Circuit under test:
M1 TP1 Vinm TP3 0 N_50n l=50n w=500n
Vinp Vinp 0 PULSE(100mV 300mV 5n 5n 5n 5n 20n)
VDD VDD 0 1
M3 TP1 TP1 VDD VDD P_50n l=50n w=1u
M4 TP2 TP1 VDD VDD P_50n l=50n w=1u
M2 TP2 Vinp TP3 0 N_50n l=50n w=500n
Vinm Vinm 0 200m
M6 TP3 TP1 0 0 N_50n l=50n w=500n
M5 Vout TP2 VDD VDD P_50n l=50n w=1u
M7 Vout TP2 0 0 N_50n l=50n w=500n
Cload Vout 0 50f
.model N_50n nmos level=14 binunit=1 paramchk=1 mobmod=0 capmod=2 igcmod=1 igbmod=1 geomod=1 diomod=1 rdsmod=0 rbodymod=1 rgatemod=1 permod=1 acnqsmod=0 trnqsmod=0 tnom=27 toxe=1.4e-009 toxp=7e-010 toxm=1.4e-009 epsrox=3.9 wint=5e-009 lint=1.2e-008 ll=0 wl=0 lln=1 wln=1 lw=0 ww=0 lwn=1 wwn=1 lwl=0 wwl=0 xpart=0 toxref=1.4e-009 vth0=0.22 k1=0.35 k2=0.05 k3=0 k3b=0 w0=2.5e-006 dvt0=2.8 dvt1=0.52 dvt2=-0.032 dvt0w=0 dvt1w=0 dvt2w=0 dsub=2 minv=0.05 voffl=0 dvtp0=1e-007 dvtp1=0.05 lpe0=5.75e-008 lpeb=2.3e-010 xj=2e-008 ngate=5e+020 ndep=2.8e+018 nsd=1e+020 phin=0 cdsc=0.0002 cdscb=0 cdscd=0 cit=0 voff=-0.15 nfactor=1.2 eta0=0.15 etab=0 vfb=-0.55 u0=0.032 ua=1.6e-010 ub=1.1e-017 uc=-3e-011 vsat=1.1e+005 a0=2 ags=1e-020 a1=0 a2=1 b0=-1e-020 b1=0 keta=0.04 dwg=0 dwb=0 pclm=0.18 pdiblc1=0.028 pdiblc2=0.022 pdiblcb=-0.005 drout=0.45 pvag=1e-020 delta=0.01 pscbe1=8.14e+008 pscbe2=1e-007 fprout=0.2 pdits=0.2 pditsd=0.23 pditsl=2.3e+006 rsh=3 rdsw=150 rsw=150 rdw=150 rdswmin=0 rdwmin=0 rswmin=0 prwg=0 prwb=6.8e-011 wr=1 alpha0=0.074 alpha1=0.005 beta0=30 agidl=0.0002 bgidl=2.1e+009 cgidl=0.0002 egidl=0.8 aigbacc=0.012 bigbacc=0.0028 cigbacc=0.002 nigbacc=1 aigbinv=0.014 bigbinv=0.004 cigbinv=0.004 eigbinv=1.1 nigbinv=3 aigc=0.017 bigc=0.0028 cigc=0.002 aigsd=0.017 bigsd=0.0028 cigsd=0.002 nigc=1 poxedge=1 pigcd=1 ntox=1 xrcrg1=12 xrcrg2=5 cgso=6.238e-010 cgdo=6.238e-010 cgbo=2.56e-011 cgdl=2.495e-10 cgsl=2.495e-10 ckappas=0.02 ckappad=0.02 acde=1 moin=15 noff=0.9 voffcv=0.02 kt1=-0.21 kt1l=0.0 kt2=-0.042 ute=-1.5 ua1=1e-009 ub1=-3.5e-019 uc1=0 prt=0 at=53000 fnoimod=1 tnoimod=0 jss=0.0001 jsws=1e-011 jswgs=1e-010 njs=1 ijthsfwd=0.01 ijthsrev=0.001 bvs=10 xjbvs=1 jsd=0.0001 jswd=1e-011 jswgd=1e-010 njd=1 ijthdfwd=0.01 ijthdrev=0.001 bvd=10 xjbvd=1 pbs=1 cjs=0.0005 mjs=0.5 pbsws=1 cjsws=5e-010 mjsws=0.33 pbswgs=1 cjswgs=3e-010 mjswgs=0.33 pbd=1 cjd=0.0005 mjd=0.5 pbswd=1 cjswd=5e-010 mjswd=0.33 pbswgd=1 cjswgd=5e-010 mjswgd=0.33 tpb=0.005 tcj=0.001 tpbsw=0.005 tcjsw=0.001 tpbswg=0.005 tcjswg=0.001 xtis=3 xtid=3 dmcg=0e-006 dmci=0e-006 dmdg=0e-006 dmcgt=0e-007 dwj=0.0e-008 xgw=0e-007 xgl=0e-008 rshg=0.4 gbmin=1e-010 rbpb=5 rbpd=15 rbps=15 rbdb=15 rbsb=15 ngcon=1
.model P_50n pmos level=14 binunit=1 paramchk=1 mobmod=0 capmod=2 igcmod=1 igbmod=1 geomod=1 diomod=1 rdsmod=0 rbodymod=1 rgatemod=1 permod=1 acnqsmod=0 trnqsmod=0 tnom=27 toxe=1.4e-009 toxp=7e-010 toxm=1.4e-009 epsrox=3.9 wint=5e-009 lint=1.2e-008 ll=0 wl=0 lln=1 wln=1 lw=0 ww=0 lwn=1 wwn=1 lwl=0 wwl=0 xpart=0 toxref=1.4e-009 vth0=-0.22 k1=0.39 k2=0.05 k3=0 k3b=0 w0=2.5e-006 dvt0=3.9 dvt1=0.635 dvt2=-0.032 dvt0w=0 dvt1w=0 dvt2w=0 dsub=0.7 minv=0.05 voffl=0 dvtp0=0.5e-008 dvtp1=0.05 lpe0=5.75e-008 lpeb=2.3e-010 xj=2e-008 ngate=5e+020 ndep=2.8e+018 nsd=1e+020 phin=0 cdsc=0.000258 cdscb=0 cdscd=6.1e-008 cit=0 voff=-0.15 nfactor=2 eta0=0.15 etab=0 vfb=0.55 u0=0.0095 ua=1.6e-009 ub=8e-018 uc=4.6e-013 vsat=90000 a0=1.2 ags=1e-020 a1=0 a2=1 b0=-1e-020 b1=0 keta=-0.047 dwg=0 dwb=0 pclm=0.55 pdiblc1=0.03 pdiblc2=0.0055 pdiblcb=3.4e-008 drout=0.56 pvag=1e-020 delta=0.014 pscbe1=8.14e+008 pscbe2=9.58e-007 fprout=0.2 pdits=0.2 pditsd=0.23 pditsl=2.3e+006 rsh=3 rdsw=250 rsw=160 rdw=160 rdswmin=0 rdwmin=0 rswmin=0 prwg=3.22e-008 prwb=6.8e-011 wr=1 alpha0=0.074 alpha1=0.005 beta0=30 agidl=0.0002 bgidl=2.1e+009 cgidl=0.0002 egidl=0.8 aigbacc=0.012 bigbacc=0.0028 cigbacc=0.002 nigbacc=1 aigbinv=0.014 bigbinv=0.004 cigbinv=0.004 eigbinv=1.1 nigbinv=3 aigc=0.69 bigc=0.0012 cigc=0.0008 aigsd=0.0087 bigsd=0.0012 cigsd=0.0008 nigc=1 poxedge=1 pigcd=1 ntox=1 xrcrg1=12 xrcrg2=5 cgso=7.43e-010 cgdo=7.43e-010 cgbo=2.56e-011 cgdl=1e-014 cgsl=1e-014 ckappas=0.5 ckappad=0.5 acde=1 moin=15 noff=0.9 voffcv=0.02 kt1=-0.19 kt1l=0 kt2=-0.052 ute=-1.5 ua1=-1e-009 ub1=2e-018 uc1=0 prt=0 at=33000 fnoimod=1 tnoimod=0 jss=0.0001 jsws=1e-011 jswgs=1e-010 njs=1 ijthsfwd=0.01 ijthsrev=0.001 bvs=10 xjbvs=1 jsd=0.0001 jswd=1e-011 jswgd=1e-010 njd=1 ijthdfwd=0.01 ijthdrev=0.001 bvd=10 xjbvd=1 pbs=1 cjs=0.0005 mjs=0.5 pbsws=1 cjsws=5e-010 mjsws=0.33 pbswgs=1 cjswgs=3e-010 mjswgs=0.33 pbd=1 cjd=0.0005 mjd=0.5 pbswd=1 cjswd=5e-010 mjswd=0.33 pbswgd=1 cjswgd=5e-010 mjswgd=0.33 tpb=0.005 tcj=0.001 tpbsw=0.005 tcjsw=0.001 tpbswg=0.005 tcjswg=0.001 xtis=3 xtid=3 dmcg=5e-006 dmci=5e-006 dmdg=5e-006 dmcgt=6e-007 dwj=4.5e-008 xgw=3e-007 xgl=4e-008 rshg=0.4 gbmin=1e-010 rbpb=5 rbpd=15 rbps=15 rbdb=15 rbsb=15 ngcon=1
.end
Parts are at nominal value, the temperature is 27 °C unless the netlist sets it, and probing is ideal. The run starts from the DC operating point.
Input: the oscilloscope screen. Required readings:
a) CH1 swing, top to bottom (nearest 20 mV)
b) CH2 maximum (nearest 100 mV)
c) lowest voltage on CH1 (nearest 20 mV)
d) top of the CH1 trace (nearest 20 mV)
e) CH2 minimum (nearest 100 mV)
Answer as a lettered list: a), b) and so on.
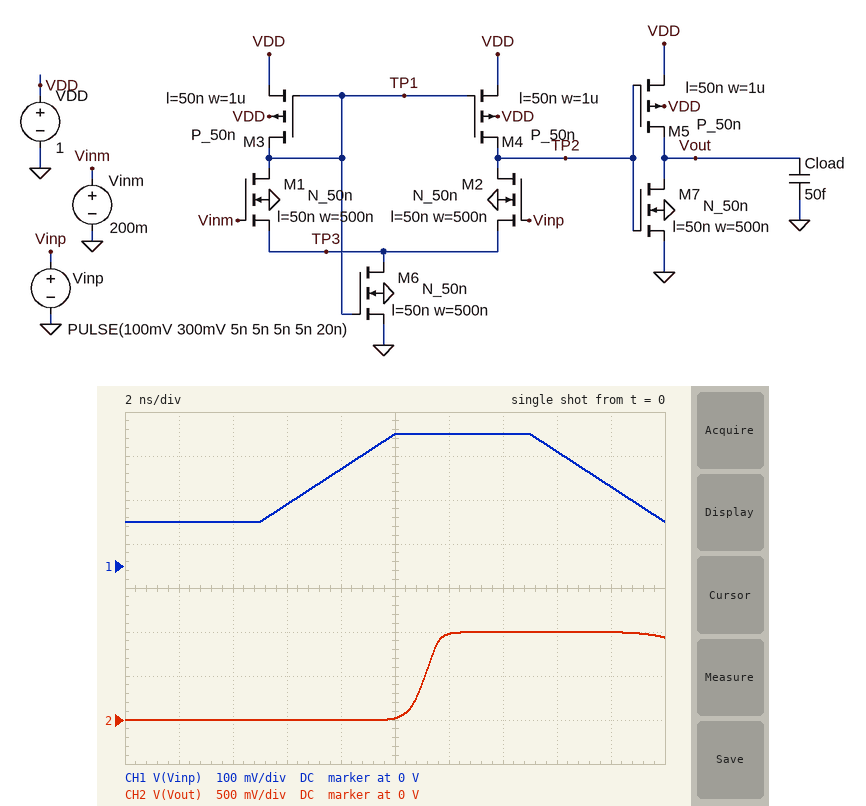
a) 200 mV
b) 1.0 V
c) 100 mV
d) 300 mV
e) 0 V
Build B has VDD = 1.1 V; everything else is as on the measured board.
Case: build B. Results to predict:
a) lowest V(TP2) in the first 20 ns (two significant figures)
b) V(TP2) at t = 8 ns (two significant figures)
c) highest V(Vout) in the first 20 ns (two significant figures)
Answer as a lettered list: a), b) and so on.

a) 110 mV
b) 1.0 V
c) 1.1 V
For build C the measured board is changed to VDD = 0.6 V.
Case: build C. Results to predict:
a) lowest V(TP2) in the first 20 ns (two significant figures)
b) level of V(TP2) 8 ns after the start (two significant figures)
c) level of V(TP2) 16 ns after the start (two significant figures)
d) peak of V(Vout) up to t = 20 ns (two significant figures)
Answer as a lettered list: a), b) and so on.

a) 17 mV
b) 560 mV
c) 25 mV
d) 600 mV
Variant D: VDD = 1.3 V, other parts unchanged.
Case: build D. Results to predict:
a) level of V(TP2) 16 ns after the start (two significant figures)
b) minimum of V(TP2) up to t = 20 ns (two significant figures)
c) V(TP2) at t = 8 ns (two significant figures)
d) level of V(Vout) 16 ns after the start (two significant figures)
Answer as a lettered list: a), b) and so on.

a) 270 mV
b) 240 mV
c) 1.2 V
d) 1.3 V
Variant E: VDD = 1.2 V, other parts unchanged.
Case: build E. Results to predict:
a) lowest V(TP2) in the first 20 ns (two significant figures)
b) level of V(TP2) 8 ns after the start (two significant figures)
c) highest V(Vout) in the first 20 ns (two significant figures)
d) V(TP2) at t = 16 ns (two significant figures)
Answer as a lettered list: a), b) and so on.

a) 170 mV
b) 1.1 V
c) 1.2 V
d) 200 mV
